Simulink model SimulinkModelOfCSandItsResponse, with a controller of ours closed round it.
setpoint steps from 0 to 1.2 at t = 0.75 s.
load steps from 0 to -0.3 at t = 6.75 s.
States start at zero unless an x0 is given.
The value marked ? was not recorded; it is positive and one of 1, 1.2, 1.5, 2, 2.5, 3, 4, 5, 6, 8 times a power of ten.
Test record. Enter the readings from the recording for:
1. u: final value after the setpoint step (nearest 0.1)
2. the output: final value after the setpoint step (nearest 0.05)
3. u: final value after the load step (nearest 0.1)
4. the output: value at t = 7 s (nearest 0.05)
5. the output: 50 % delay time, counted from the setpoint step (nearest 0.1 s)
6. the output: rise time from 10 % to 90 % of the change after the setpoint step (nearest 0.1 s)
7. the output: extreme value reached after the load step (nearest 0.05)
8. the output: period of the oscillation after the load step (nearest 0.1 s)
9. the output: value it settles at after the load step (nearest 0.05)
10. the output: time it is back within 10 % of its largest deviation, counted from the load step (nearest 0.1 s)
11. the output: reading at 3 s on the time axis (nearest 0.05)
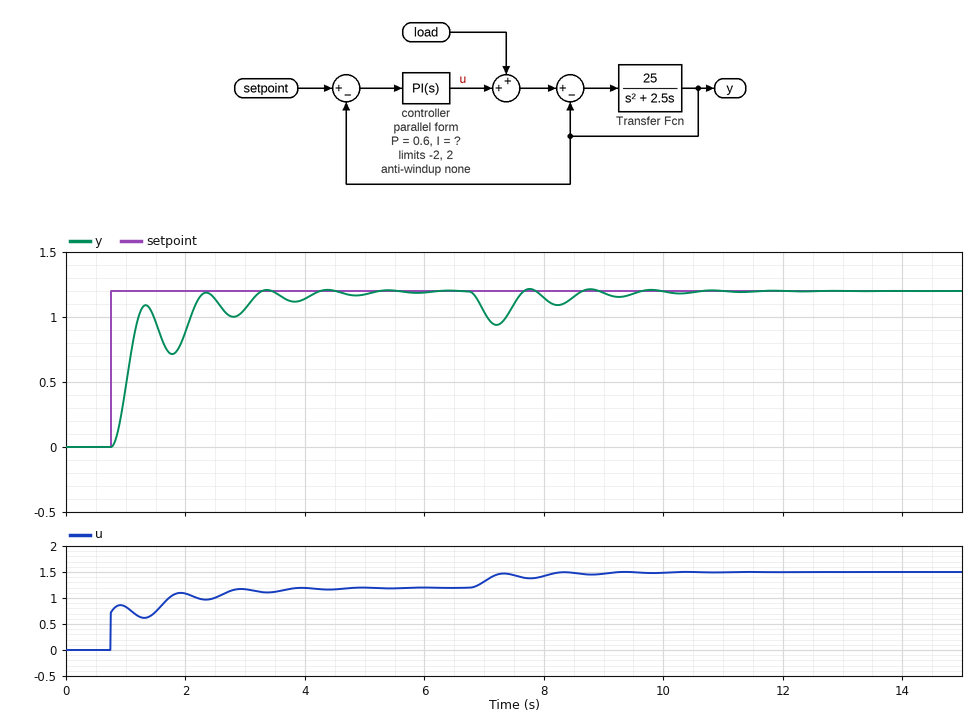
1.2
1.20
1.5
1.05
0.3 s
0.4 s
0.95
1.0 s
1.20
2.7 s
1.05
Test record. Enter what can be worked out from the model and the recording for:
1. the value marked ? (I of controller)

1.5
